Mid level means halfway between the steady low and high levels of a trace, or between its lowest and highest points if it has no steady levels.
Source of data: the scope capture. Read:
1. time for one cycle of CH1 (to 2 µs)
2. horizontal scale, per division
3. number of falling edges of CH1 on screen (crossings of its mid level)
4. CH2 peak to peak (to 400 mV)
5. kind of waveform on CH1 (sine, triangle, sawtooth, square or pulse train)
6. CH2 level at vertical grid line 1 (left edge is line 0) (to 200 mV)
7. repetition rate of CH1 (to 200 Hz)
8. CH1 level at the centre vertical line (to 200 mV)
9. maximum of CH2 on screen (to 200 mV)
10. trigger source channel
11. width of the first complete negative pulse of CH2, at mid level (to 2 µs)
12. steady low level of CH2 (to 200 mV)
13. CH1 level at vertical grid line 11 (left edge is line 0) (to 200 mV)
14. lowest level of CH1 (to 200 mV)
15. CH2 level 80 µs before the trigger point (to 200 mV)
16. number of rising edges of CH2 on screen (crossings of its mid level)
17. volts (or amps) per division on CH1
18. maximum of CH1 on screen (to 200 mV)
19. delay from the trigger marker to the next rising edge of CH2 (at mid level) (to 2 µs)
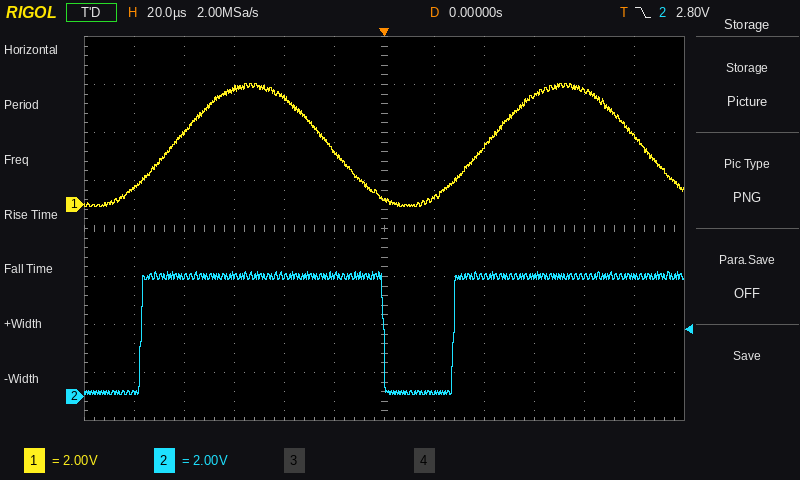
124 µs
20 µs
2
5.2 V
sine
200 mV
8.0 kHz
200 mV
5.2 V
CH2
28 µs
200 mV
2.8 V
0.0 V
5.0 V
2
2 V
5.0 V
28 µs
